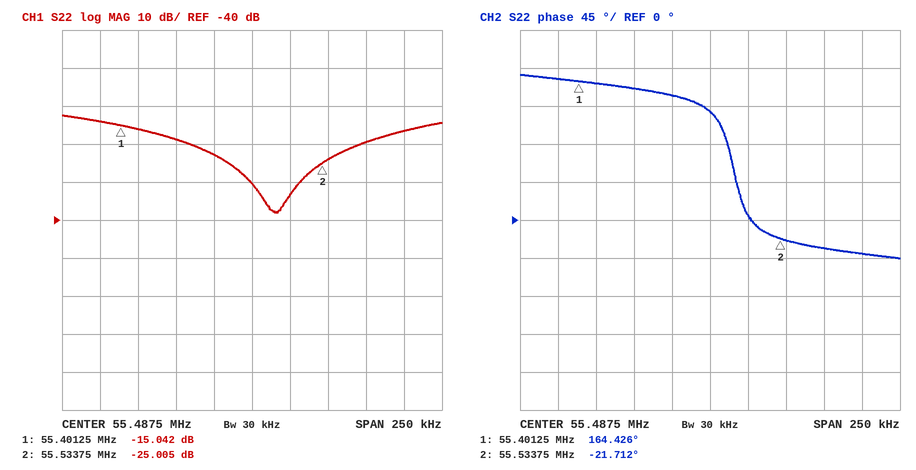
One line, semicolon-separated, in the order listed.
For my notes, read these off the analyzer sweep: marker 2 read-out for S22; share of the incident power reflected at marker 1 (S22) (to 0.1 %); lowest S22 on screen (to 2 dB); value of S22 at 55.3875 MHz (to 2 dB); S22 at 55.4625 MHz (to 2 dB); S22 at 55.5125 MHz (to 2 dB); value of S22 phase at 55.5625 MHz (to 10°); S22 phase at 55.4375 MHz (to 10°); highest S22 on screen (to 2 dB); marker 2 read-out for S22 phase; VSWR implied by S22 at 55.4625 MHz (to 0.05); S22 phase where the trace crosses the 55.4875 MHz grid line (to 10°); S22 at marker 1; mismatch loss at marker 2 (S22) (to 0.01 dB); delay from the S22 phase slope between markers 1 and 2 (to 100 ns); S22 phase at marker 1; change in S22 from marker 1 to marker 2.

-25.005 dB; 3.1 %; -38 dB; -14 dB; -22 dB; -34 dB; -30°; 160°; -12 dB; -21.712°; 1.15; 130°; -15.042 dB; 0.01 dB; 3.9 µs; 164.426°; -9.963 dB
